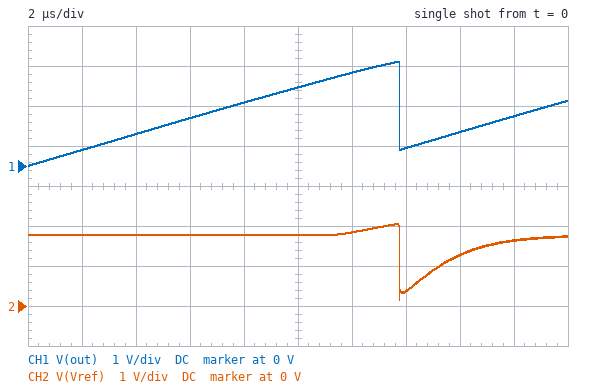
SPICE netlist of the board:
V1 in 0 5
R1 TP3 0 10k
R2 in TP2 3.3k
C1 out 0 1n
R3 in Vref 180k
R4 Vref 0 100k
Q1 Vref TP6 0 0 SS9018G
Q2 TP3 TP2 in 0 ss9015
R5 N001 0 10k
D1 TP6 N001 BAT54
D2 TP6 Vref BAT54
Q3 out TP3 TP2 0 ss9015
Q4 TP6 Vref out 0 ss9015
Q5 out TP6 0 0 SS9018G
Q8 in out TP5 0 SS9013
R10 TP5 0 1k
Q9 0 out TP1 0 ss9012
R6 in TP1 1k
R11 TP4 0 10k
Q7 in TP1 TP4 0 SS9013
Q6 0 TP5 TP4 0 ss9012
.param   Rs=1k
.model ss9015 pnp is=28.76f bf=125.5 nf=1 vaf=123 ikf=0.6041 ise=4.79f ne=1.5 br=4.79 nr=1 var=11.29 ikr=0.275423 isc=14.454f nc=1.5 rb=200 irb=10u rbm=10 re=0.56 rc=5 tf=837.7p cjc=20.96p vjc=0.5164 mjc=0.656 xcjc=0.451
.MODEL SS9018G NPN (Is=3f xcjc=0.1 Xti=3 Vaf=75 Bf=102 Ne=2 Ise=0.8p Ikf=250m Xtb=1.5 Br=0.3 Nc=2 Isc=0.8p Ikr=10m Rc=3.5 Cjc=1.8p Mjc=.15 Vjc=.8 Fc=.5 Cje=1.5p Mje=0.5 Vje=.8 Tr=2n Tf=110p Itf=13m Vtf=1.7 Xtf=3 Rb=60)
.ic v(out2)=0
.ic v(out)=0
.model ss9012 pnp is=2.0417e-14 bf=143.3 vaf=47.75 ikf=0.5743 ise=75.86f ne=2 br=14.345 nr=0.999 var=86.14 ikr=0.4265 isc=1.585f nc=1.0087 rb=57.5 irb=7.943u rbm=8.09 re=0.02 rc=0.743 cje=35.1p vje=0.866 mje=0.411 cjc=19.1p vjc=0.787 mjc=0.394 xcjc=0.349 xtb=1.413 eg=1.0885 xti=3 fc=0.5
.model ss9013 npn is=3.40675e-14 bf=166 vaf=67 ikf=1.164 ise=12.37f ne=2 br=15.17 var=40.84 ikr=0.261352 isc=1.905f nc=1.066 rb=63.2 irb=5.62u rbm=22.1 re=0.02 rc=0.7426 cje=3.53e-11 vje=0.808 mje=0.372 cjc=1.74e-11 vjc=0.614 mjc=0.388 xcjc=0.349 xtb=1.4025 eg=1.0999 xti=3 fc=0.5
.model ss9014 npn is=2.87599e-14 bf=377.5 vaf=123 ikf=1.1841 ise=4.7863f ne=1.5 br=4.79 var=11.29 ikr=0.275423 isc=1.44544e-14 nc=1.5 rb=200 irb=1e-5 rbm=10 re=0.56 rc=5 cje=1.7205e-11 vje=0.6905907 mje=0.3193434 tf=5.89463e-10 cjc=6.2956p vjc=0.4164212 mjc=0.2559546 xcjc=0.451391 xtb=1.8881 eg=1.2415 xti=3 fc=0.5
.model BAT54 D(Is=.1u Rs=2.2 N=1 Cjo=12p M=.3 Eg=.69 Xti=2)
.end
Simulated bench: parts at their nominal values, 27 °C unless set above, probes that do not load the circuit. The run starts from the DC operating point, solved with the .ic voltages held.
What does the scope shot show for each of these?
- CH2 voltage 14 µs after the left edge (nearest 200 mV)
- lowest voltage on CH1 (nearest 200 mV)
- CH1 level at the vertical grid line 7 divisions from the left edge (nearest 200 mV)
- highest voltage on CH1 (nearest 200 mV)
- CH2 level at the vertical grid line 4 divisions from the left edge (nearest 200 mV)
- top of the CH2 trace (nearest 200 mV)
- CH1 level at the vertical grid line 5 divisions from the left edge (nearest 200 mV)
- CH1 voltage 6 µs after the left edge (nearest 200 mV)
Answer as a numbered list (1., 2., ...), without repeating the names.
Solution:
1. 400 mV
2. 0 V
3. 400 mV
4. 2.6 V
5. 1.8 V
6. 2.0 V
7. 2.0 V
8. 1.2 V
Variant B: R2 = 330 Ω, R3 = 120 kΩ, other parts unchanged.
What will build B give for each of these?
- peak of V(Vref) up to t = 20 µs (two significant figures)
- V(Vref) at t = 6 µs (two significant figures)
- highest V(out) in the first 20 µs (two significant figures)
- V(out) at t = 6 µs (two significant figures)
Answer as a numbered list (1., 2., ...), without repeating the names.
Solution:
1. 2.7 V
2. 450 mV
3. 3.3 V
4. 1.1 V
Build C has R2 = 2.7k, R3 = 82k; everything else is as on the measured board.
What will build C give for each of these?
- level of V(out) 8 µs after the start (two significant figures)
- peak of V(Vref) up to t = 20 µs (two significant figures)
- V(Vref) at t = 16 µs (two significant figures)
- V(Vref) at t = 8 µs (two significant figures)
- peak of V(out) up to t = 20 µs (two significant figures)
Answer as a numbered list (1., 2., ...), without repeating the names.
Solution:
1. 1.9 V
2. 3.0 V
3. 570 mV
4. 2.7 V
5. 3.5 V
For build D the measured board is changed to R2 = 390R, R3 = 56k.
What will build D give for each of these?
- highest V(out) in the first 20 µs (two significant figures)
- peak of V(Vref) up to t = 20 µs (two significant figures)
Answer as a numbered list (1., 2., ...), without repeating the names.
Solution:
1. 4.2 V
2. 3.6 V
